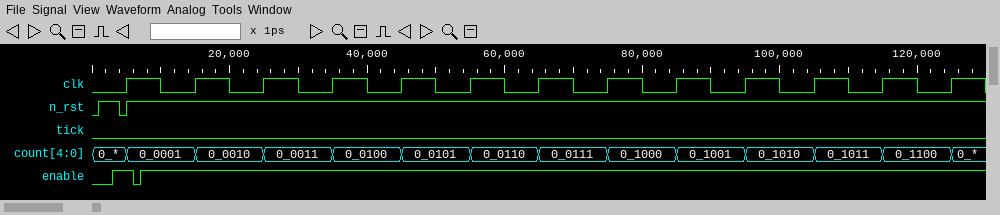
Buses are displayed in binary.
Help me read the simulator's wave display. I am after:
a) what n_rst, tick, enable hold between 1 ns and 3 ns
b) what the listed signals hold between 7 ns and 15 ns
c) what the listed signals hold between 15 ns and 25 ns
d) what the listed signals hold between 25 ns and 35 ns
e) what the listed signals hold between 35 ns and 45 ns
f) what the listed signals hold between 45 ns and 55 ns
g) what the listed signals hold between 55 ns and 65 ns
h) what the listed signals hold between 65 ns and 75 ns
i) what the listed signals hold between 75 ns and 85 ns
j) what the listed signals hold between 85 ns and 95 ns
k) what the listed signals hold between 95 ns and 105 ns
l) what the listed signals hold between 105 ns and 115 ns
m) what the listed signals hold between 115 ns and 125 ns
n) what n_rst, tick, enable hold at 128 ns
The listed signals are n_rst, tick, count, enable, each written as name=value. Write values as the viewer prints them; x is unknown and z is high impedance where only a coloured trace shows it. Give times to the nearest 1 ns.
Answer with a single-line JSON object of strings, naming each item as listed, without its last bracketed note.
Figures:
{"what n_rst, tick, enable hold between 1 ns and 3 ns": "n_rst=1, tick=0, enable=0", "what the listed signals hold between 7 ns and 15 ns": "n_rst=1, tick=0, count=0_0001, enable=1", "what the listed signals hold between 15 ns and 25 ns": "n_rst=1, tick=0, count=0_0010, enable=1", "what the listed signals hold between 25 ns and 35 ns": "n_rst=1, tick=0, count=0_0011, enable=1", "what the listed signals hold between 35 ns and 45 ns": "n_rst=1, tick=0, count=0_0100, enable=1", "what the listed signals hold between 45 ns and 55 ns": "n_rst=1, tick=0, count=0_0101, enable=1", "what the listed signals hold between 55 ns and 65 ns": "n_rst=1, tick=0, count=0_0110, enable=1", "what the listed signals hold between 65 ns and 75 ns": "n_rst=1, tick=0, count=0_0111, enable=1", "what the listed signals hold between 75 ns and 85 ns": "n_rst=1, tick=0, count=0_1000, enable=1", "what the listed signals hold between 85 ns and 95 ns": "n_rst=1, tick=0, count=0_1001, enable=1", "what the listed signals hold between 95 ns and 105 ns": "n_rst=1, tick=0, count=0_1010, enable=1", "what the listed signals hold between 105 ns and 115 ns": "n_rst=1, tick=0, count=0_1011, enable=1", "what the listed signals hold between 115 ns and 125 ns": "n_rst=1, tick=0, count=0_1100, enable=1", "what n_rst, tick, enable hold at 128 ns": "n_rst=1, tick=0, enable=1"}
